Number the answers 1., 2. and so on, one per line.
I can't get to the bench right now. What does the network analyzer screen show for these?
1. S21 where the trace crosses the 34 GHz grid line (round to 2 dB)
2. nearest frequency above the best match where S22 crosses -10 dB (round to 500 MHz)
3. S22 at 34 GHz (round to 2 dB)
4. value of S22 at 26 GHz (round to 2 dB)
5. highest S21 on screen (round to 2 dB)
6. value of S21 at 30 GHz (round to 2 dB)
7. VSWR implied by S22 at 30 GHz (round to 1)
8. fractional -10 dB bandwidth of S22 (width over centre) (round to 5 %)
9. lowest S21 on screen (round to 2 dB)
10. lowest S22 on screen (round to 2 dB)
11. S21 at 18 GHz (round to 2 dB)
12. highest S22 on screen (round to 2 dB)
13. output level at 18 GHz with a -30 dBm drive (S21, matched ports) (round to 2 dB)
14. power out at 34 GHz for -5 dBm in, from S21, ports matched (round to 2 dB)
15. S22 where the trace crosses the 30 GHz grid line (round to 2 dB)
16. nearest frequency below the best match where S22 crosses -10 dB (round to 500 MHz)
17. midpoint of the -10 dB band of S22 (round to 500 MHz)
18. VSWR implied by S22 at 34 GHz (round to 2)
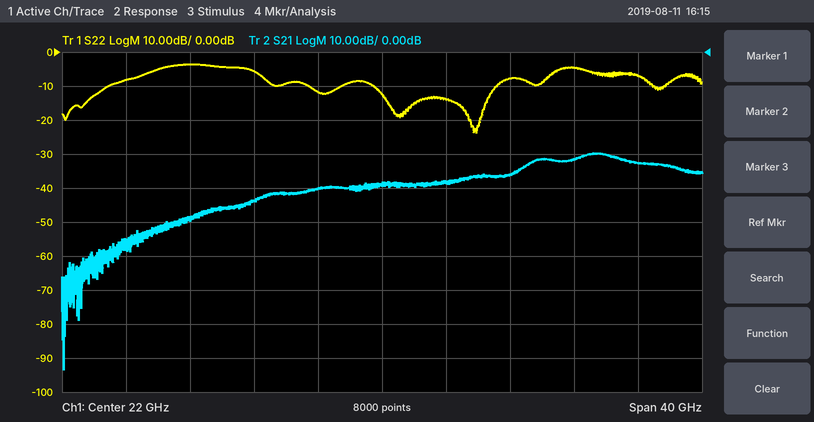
1. -32 dB
2. 29.0 GHz
3. -4 dB
4. -14 dB
5. -30 dB
6. -36 dB
7. 2
8. 30 %
9. -94 dB
10. -24 dB
11. -40 dB
12. -4 dB
13. -70 dBm
14. -36 dBm
15. -8 dB
16. 21.5 GHz
17. 25.5 GHz
18. 4
